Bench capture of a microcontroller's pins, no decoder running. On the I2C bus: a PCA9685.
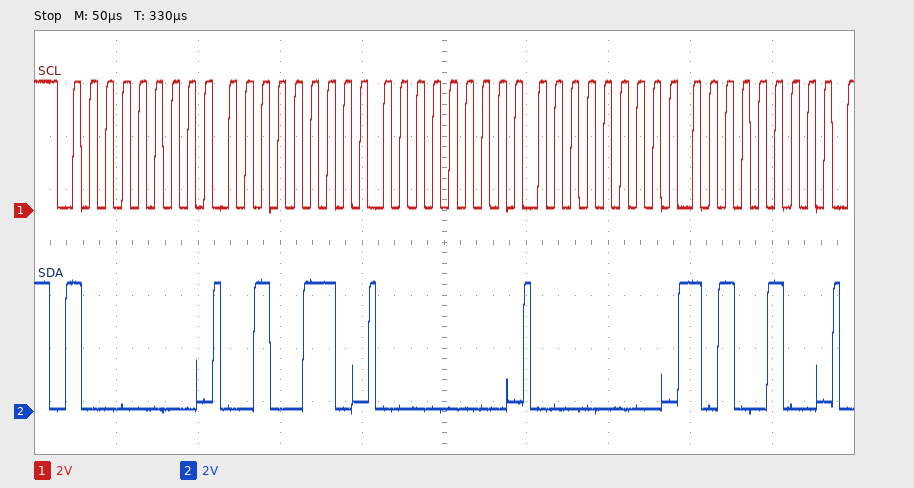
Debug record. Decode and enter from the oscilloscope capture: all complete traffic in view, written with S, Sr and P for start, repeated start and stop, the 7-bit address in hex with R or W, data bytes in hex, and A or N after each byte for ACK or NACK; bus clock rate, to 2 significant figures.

S 40W A 26 A 00 A 00 A A4 A
100 kHz
